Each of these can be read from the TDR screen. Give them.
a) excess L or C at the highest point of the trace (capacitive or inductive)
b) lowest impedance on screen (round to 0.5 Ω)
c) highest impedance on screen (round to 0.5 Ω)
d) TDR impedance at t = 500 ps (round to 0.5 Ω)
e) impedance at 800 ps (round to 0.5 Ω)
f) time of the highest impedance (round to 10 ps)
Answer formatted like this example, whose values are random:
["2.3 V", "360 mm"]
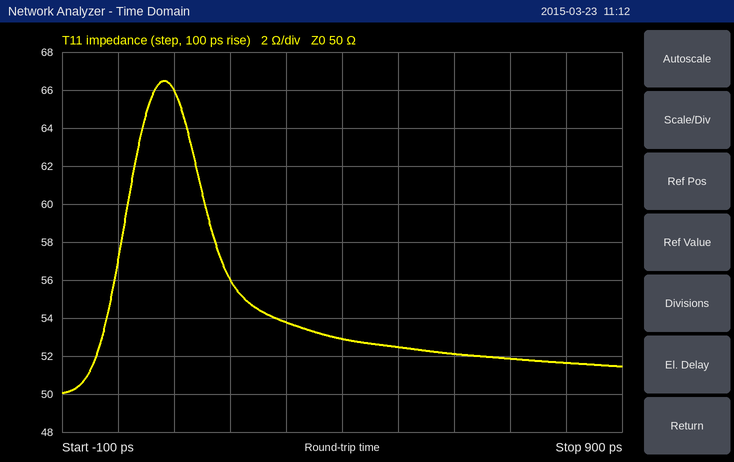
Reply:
["inductive", "50.0 Ω", "66.5 Ω", "52.5 Ω", "51.5 Ω", "80 ps"]
